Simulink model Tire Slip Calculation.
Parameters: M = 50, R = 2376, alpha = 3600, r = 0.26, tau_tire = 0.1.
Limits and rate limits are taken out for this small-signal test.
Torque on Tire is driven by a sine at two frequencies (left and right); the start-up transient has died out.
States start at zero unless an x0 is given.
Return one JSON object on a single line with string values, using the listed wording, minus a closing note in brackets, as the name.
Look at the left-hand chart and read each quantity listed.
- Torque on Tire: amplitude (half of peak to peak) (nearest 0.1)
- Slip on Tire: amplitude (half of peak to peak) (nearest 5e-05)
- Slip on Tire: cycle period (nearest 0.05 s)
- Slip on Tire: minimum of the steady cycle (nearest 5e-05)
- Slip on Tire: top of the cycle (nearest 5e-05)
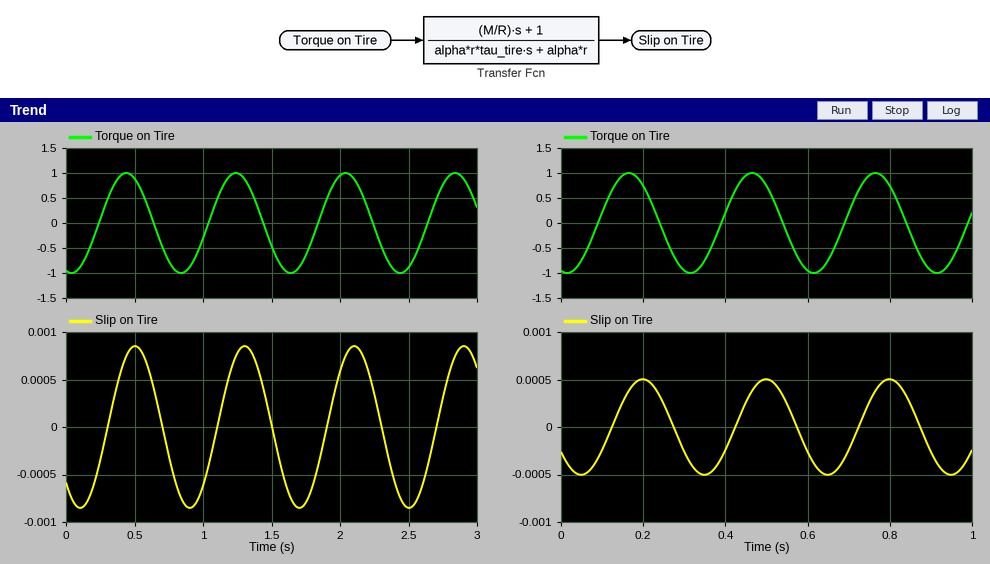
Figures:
{"Torque on Tire: amplitude (half of peak to peak)": "1.0", "Slip on Tire: amplitude (half of peak to peak)": "0.00085", "Slip on Tire: cycle period": "0.80 s", "Slip on Tire: minimum of the steady cycle": "-0.00085", "Slip on Tire: top of the cycle": "0.00085"}
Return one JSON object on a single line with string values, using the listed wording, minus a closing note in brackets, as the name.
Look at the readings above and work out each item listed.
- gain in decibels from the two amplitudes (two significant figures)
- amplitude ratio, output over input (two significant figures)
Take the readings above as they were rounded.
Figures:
{"gain in decibels from the two amplitudes": "-61 dB", "amplitude ratio, output over input": "0.00085"}
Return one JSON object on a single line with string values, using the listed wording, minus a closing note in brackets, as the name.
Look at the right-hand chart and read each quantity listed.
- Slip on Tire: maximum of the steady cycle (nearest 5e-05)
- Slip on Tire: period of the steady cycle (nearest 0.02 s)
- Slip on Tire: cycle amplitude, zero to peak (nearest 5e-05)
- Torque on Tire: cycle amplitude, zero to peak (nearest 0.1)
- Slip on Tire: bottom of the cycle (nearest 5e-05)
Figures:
{"Slip on Tire: maximum of the steady cycle": "0.00050", "Slip on Tire: period of the steady cycle": "0.30 s", "Slip on Tire: cycle amplitude, zero to peak": "0.00050", "Torque on Tire: cycle amplitude, zero to peak": "1.0", "Slip on Tire: bottom of the cycle": "-0.00050"}
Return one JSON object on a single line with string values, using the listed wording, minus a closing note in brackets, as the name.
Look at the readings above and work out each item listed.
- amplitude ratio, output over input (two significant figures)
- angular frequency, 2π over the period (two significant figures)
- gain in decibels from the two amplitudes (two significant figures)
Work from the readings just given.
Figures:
{"amplitude ratio, output over input": "0.00050", "angular frequency, 2π over the period": "21 rad/s", "gain in decibels from the two amplitudes": "-66 dB"}
